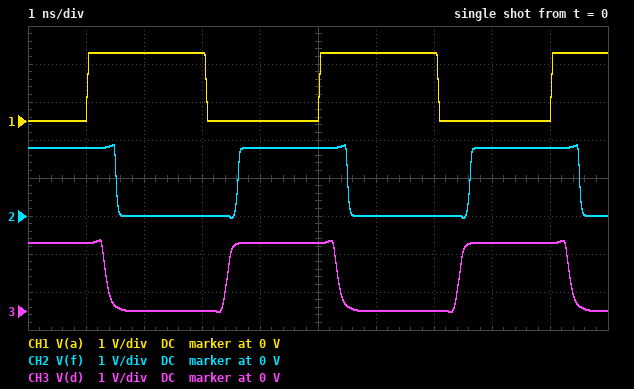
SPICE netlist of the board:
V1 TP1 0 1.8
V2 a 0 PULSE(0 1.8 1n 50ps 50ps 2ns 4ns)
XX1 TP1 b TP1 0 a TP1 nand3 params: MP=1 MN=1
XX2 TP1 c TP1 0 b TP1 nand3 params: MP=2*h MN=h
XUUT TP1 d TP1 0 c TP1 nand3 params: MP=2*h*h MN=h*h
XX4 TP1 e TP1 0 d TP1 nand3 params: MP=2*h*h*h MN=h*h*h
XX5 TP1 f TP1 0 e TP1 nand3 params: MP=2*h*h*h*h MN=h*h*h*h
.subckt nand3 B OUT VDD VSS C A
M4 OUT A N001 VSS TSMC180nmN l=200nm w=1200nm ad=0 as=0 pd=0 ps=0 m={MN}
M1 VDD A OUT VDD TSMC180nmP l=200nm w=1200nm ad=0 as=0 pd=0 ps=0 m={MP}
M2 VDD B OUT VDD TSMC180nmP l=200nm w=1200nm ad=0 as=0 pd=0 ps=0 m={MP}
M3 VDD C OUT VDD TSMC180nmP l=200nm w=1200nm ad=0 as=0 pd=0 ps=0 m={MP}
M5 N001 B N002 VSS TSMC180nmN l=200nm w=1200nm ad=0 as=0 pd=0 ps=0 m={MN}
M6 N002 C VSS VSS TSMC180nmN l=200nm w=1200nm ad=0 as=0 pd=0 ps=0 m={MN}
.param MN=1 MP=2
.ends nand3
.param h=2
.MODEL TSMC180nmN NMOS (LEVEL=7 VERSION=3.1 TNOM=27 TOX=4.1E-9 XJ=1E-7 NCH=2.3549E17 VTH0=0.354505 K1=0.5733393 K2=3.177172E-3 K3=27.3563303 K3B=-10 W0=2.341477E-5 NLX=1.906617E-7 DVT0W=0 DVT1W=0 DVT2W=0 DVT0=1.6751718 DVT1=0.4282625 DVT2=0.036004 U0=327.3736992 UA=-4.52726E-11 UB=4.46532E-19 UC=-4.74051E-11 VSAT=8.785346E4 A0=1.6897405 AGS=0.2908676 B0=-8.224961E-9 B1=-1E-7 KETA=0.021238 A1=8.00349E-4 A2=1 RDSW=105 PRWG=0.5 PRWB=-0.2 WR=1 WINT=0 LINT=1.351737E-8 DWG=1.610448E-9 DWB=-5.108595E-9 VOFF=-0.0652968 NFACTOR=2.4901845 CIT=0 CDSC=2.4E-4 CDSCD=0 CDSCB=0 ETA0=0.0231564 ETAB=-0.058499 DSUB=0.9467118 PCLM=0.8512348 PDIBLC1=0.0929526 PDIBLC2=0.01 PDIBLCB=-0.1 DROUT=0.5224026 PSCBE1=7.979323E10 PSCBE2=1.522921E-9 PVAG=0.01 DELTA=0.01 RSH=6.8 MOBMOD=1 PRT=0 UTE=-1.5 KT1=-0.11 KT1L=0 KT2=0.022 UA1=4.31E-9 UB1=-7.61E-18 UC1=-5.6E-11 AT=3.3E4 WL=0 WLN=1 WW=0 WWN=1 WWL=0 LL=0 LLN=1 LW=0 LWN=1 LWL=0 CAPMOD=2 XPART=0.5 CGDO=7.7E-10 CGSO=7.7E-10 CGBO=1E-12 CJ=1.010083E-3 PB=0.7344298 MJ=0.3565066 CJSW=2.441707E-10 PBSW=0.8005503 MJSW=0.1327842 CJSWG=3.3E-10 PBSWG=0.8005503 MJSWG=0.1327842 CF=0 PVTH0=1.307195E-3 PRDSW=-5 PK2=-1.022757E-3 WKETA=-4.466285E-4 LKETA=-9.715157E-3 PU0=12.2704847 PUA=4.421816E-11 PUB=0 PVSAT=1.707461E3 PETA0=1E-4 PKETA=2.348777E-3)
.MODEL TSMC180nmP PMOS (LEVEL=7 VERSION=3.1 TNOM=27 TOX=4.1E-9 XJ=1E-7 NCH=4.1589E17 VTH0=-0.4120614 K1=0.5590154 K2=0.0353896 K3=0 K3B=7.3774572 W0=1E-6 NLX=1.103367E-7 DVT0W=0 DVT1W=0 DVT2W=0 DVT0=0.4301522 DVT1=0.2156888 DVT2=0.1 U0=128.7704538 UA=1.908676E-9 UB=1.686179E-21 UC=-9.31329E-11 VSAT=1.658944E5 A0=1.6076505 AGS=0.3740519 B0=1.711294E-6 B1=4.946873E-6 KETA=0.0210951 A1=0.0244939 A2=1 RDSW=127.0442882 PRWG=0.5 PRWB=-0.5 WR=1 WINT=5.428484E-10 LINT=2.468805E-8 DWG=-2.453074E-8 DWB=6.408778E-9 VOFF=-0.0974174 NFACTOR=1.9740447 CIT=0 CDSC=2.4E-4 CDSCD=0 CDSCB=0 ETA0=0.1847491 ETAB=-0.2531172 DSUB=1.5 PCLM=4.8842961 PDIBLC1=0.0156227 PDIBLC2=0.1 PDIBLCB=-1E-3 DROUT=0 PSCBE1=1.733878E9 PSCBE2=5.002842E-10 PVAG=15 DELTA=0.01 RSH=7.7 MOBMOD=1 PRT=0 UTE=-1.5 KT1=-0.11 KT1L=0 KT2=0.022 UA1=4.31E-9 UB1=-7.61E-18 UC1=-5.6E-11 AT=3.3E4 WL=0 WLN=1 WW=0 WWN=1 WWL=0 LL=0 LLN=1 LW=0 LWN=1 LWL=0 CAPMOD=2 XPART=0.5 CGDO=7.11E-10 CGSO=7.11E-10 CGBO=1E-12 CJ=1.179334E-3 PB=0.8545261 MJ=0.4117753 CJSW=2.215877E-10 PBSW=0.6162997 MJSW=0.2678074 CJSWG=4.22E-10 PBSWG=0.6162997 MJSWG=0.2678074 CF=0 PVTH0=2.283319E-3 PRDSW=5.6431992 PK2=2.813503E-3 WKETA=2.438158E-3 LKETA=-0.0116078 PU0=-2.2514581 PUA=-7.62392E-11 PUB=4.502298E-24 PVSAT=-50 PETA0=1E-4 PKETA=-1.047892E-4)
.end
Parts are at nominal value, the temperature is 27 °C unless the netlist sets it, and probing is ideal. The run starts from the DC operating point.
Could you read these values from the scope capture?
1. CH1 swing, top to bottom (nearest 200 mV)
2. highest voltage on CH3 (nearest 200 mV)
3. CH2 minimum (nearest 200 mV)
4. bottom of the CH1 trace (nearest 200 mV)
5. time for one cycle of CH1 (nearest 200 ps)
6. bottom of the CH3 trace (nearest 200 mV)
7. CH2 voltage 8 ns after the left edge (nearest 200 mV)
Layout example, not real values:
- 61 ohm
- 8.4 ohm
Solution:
- 1.8 V
- 1.8 V
- 0 V
- 0 V
- 4.0 ns
- 0 V
- 1.8 V
